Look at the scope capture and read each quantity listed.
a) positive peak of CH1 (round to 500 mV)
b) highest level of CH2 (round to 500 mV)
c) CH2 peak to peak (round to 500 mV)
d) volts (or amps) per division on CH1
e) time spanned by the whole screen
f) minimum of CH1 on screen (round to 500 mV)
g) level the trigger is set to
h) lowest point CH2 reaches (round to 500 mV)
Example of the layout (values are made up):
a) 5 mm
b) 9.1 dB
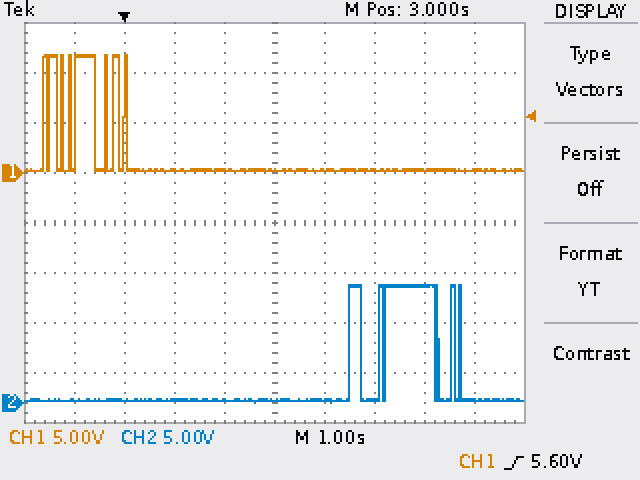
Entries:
a) 12.0 V
b) 12.0 V
c) 12.0 V
d) 5 V
e) 10 s
f) 0.0 V
g) 5.60 V
h) 0.0 V
